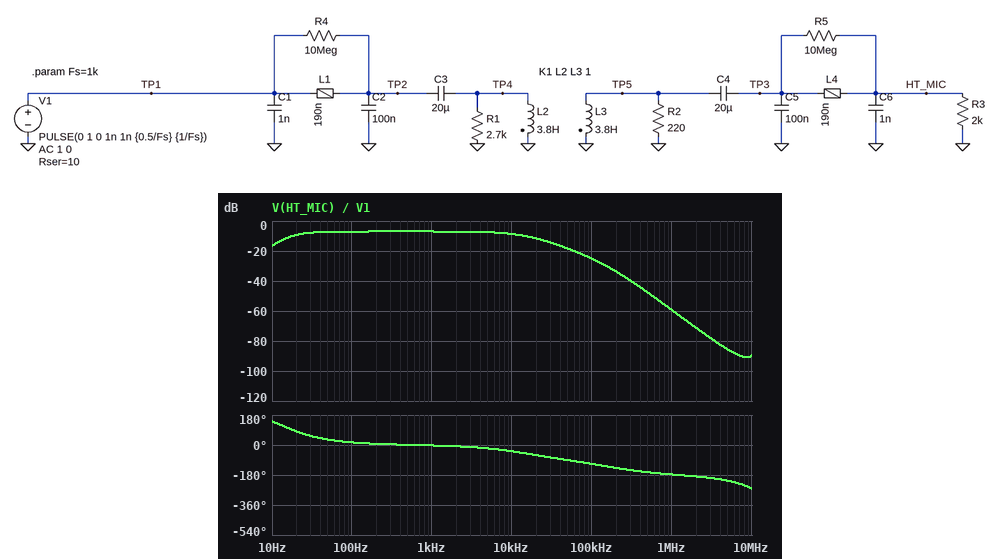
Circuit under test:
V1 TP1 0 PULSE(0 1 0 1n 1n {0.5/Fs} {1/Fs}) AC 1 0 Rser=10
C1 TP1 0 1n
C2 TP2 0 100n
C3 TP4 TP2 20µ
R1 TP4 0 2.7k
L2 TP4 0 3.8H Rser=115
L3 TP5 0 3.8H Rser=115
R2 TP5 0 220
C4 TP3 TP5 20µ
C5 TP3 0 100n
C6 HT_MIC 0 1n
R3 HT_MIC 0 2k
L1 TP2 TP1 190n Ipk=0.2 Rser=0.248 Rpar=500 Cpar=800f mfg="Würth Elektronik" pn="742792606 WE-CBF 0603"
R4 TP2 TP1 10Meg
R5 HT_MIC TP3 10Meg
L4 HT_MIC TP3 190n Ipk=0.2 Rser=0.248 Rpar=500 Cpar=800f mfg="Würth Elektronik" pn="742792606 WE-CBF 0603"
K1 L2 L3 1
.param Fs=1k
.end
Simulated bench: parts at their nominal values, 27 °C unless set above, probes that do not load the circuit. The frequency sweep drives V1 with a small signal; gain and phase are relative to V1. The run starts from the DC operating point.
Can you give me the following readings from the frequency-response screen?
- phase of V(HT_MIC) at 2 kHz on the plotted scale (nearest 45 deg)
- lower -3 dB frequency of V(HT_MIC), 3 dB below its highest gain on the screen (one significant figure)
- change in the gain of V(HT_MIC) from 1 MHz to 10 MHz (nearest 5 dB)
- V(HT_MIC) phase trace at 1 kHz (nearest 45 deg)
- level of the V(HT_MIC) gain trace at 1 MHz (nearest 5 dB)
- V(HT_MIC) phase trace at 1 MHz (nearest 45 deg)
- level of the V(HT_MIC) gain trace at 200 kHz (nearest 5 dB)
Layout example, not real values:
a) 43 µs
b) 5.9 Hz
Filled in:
a) 0 deg
b) 20 Hz
c) -30 dB
d) 0 deg
e) -60 dB
f) -180 deg
g) -35 dB
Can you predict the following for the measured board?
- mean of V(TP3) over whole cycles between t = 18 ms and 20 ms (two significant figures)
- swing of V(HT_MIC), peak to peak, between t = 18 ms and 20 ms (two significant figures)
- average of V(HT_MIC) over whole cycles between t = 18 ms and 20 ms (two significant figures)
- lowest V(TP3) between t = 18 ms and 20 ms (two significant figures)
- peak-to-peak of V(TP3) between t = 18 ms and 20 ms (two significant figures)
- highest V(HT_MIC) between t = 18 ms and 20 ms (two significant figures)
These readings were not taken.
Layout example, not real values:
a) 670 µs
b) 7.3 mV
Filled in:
a) -51 mV
b) 460 mV
c) -51 mV
d) -280 mV
e) 460 mV
f) 180 mV
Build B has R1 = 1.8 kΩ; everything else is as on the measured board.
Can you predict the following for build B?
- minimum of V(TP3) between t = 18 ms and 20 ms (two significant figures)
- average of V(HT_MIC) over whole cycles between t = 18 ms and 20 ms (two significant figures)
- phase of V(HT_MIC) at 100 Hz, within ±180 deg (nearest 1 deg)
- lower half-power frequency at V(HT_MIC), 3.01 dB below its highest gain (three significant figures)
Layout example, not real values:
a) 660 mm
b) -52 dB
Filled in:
a) -280 mV
b) -48 mV
c) 17 deg
d) 19.2 Hz
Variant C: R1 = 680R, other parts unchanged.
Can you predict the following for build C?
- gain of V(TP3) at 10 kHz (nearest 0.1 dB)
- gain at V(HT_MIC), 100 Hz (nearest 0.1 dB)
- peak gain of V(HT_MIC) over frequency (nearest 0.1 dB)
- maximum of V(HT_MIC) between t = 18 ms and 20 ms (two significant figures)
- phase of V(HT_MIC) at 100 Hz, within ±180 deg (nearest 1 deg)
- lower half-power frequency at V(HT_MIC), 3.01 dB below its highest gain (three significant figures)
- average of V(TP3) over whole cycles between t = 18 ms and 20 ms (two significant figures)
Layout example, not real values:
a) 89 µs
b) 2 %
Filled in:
a) -8.8 dB
b) -7.3 dB
c) -7.1 dB
d) 190 mV
e) 20 deg
f) 25.8 Hz
g) -38 mV
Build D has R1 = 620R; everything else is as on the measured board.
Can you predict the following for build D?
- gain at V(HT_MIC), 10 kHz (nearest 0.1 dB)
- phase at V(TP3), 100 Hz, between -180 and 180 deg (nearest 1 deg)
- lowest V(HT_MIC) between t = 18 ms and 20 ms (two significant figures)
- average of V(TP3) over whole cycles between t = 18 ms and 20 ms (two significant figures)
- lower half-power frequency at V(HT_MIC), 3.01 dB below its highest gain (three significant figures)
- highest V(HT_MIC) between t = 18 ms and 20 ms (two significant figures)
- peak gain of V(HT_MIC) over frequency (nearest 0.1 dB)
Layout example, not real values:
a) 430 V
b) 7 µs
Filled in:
a) -8.8 dB
b) 21 deg
c) -270 mV
d) -37 mV
e) 26.9 Hz
f) 190 mV
g) -7.1 dB
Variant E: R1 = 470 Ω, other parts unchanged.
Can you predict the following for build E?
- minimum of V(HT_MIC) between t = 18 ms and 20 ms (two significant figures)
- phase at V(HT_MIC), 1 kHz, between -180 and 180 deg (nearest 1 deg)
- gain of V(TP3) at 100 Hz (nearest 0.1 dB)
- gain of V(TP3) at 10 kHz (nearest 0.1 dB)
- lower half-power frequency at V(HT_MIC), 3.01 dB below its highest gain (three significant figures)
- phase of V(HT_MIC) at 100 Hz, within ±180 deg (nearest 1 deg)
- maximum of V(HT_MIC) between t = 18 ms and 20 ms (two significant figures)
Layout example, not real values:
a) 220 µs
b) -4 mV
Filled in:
a) -260 mV
b) -2 deg
c) -7.5 dB
d) -8.8 dB
e) 30.8 Hz
f) 23 deg
g) 200 mV
